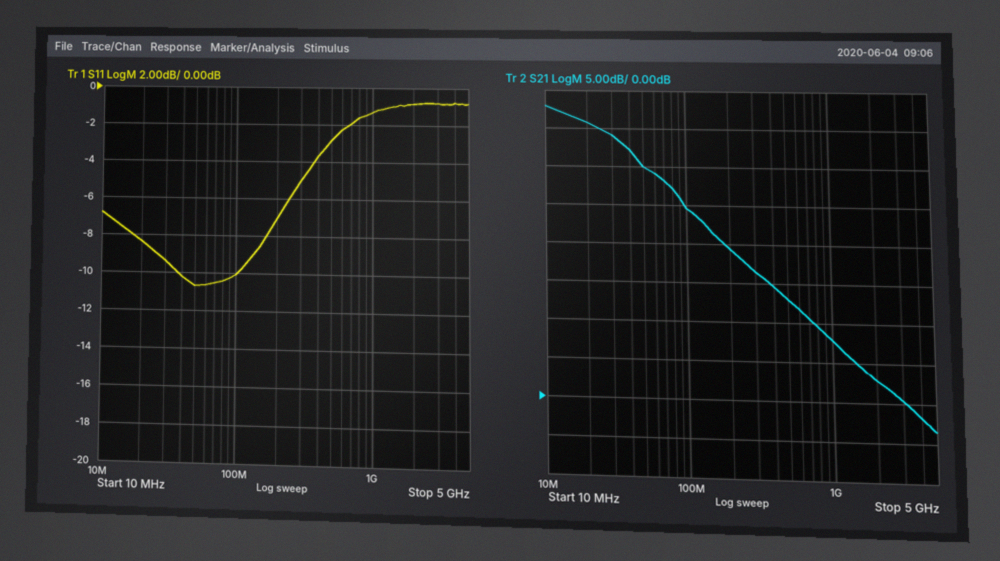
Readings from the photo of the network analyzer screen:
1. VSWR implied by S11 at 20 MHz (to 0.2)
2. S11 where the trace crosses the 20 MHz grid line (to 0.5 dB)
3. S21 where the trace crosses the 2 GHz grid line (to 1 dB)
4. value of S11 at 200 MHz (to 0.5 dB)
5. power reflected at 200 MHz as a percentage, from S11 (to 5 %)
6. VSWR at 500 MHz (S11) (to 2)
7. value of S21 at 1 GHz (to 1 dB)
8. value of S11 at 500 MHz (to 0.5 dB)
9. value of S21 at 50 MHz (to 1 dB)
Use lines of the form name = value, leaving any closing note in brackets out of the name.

VSWR implied by S11 at 20 MHz = 2.2
S11 where the trace crosses the 20 MHz grid line = -8.5 dB
S21 where the trace crosses the 2 GHz grid line = 3 dB
value of S11 at 200 MHz = -7.0 dB
power reflected at 200 MHz as a percentage, from S11 = 20 %
VSWR at 500 MHz (S11) = 6
value of S21 at 1 GHz = 8 dB
value of S11 at 500 MHz = -3.0 dB
value of S21 at 50 MHz = 30 dB
